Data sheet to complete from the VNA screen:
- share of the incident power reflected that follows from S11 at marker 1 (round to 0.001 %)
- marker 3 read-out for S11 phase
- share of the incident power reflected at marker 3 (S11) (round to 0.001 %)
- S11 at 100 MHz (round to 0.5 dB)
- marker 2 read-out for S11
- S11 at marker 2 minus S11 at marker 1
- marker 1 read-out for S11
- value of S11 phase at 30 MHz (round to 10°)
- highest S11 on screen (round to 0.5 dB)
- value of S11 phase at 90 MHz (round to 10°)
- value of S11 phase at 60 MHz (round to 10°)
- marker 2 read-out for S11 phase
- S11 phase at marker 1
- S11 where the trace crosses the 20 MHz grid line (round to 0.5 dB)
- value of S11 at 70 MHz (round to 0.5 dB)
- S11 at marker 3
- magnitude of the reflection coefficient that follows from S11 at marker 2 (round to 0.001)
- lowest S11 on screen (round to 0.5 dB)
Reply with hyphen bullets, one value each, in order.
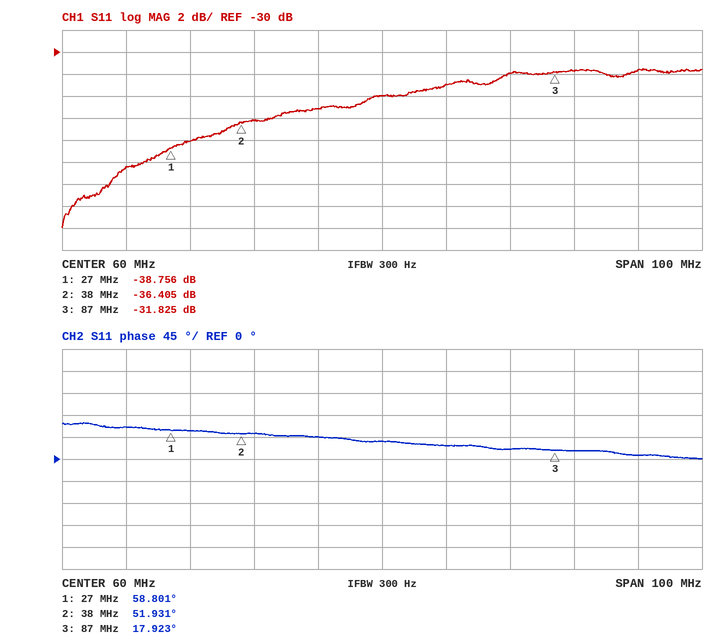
- 0.013 %
- 17.923°
- 0.066 %
- -31.5 dB
- -36.405 dB
- 2.351 dB
- -38.756 dB
- 60°
- -31.5 dB
- 20°
- 40°
- 51.931°
- 58.801°
- -40.5 dB
- -33.0 dB
- -31.825 dB
- 0.015
- -46.0 dB
